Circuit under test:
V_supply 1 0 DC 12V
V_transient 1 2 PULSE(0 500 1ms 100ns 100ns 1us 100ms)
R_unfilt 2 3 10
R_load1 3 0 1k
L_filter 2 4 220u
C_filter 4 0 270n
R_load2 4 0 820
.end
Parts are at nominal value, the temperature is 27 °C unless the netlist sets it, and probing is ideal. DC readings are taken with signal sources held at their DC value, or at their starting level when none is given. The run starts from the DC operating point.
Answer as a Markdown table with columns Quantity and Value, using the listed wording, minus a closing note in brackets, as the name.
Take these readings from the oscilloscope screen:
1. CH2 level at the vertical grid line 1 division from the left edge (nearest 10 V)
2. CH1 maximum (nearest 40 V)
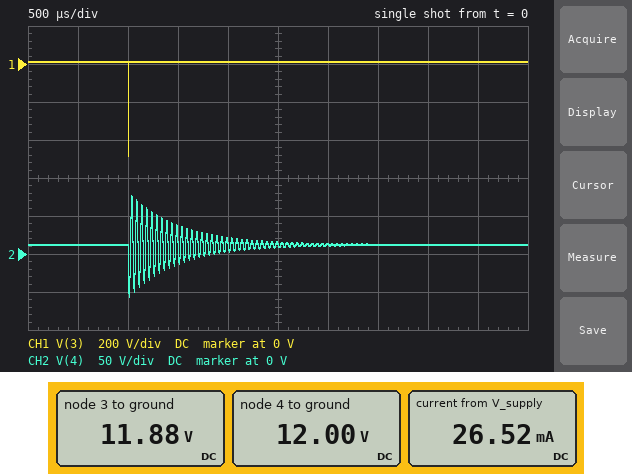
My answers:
| Quantity | Value |
|---|---|
| CH2 level at the vertical grid line 1 division from the left edge | 10 V |
| CH1 maximum | 0 V |
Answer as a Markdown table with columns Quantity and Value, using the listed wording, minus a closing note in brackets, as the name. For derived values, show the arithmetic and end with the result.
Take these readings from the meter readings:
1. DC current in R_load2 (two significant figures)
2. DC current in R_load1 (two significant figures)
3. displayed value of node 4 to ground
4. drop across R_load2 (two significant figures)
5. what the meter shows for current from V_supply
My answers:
| Quantity | Value |
|---|---|
| DC current in R_load2 | (12 V) / 820 Ω = 15 mA |
| DC current in R_load1 | (11.88 V) / 1 kΩ = 12 mA |
| displayed value of node 4 to ground | 12.00 V |
| drop across R_load2 | 12 V = 12 V |
| what the meter shows for current from V_supply | 26.52 mA |
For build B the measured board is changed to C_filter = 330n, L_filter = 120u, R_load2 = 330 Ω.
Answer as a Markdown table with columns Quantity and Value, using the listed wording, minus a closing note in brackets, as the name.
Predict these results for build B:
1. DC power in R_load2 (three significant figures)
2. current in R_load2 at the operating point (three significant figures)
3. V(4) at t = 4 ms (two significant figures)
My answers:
| Quantity | Value |
|---|---|
| DC power in R_load2 | 436 mW |
| current in R_load2 at the operating point | 36.4 mA |
| V(4) at t = 4 ms | 12 V |
